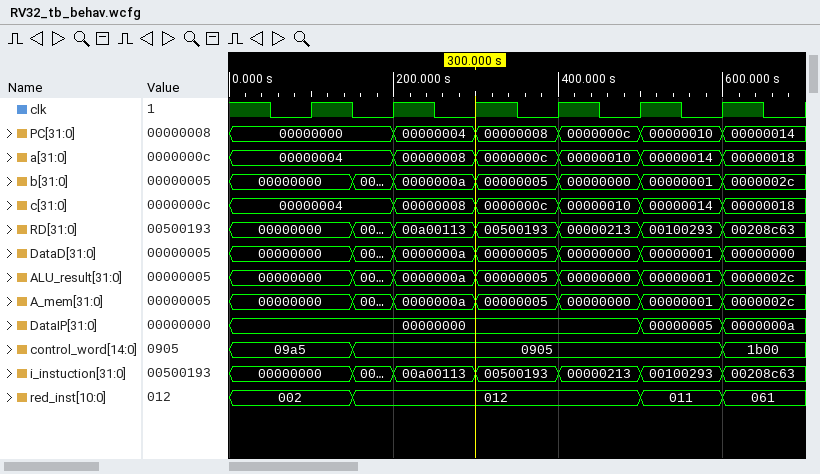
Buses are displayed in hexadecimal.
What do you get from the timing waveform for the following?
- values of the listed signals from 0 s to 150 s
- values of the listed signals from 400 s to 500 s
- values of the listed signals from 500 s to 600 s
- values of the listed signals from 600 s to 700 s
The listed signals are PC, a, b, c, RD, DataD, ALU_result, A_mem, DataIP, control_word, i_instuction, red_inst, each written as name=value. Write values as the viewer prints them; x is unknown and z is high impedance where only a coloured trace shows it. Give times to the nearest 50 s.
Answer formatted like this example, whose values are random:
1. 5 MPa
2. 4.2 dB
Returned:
1. PC=00000000, a=00000004, b=00000000, c=00000004, RD=00000000, DataD=00000000, ALU_result=00000000, A_mem=00000000, DataIP=00000000, control_word=09a5, i_instuction=00000000, red_inst=002
2. PC=0000000c, a=00000010, b=00000000, c=00000010, RD=00000213, DataD=00000000, ALU_result=00000000, A_mem=00000000, DataIP=00000000, control_word=0905, i_instuction=00000213, red_inst=012
3. PC=00000010, a=00000014, b=00000001, c=00000014, RD=00100293, DataD=00000001, ALU_result=00000001, A_mem=00000001, DataIP=00000005, control_word=0905, i_instuction=00100293, red_inst=011
4. PC=00000014, a=00000018, b=0000002c, c=00000018, RD=00208c63, DataD=00000000, ALU_result=0000002c, A_mem=0000002c, DataIP=0000000a, control_word=1b00, i_instuction=00208c63, red_inst=061
